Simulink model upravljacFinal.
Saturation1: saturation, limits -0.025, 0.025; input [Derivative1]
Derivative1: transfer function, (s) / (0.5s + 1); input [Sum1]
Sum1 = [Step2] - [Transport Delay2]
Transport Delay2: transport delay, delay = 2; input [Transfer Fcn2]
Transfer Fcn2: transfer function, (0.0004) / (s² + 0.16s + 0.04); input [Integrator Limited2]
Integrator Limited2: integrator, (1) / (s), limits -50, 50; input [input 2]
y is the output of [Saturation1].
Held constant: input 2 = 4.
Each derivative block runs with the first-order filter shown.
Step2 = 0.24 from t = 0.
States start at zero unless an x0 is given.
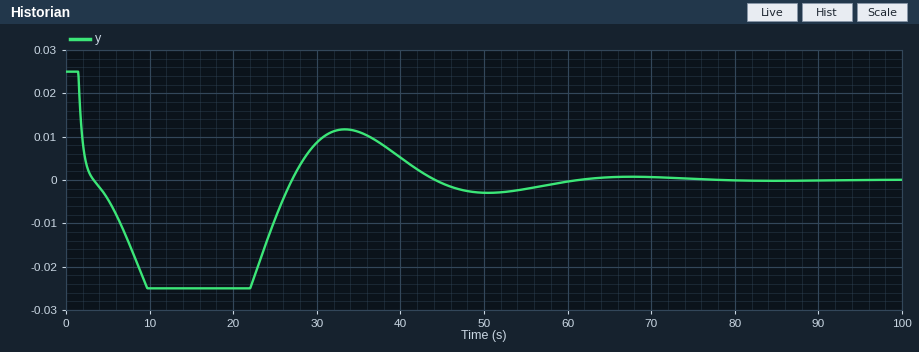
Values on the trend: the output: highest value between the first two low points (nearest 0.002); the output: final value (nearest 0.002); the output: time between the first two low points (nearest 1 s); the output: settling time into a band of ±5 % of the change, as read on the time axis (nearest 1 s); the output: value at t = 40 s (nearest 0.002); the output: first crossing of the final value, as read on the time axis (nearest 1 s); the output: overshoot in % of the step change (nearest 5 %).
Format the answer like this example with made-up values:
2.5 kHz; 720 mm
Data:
0.012; 0.000; 35 s; 57 s; 0.006; 3 s; 100 %
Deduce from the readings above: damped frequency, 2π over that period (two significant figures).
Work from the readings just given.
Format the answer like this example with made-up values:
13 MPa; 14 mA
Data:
0.18 rad/s
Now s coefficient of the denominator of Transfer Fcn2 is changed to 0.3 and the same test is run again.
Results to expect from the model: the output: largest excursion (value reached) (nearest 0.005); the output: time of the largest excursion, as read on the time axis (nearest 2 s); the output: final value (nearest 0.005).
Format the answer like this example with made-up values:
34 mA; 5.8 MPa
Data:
-0.025; 12 s; 0.000
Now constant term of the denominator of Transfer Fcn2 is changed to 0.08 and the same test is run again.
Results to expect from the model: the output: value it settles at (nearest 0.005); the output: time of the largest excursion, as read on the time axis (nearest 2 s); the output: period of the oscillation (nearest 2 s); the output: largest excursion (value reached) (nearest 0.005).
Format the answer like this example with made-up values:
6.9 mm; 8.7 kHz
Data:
0.000; 12 s; 24 s; -0.025
